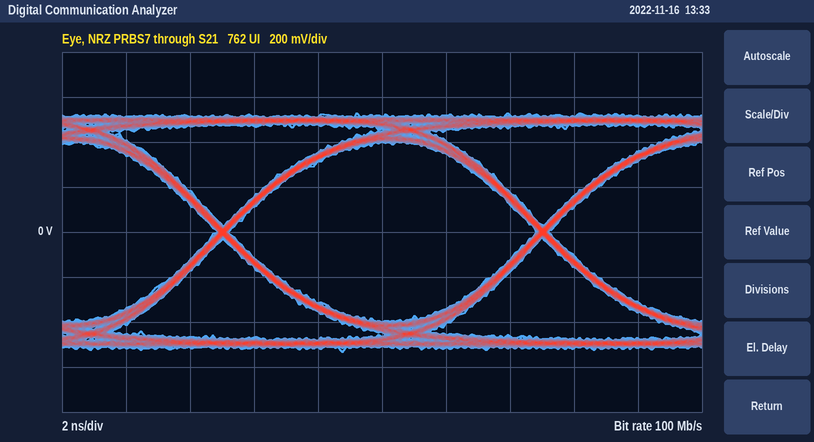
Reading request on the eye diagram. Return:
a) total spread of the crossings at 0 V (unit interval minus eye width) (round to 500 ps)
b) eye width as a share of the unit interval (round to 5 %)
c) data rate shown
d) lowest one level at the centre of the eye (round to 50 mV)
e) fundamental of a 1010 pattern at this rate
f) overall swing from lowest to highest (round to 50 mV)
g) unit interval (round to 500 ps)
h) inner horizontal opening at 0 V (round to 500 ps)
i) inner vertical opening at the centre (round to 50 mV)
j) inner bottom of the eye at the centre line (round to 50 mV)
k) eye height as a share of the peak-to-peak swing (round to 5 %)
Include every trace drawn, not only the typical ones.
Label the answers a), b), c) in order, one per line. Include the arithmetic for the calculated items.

a) 500 ps
b) 9.5 ns / 10.0 ns ≈ 95 %
c) 100 Mb/s
d) 400 mV
e) 50 MHz
f) 1.05 V
g) 10.0 ns
h) 9.5 ns
i) 800 mV
j) -400 mV
k) 800 mV / 1.05 V ≈ 76.2 %, so 75 % to the nearest 5 %
